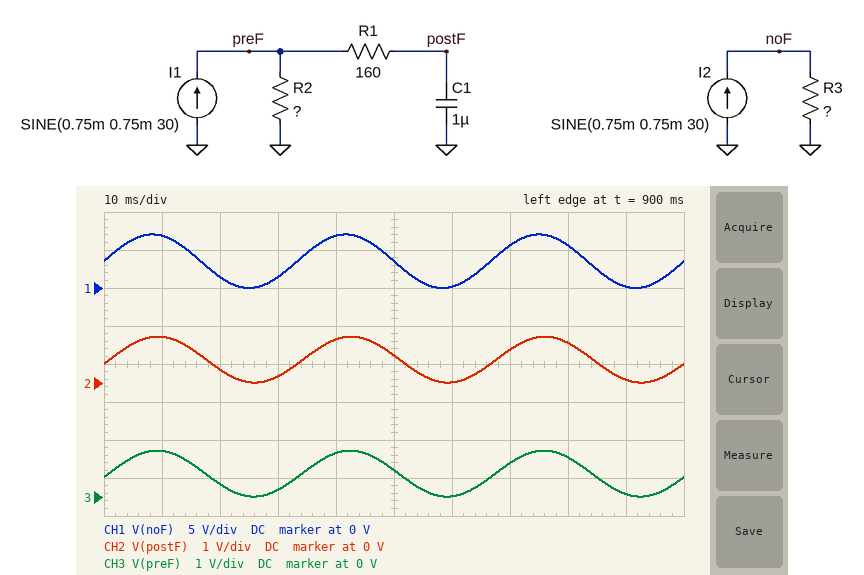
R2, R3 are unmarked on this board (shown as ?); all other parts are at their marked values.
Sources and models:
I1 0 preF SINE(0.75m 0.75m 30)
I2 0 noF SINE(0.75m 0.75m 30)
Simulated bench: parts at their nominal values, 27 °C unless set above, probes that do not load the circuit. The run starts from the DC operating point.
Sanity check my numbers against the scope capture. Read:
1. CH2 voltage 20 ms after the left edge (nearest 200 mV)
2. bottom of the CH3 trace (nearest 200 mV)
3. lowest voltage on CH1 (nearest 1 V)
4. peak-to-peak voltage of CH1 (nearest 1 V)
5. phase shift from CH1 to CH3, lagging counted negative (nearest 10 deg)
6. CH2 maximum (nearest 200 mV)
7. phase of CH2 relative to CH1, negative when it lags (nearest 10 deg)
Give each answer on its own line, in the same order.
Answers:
400 mV
0 V
0 V
7 V
-10 deg
1.2 V
-10 deg
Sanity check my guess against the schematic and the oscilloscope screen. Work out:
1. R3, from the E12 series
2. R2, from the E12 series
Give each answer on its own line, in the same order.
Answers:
4.7 kΩ
820 Ω
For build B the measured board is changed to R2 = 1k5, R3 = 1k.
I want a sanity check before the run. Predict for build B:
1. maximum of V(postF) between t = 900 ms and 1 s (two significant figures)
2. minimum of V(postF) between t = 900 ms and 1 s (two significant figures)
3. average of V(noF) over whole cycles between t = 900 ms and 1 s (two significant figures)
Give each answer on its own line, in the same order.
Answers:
2.2 V
51 mV
750 mV
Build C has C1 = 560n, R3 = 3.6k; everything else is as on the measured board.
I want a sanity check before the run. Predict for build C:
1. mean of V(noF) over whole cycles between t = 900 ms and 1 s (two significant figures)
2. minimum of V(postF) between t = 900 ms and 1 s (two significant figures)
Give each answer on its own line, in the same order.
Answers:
2.7 V
3.3 mV
